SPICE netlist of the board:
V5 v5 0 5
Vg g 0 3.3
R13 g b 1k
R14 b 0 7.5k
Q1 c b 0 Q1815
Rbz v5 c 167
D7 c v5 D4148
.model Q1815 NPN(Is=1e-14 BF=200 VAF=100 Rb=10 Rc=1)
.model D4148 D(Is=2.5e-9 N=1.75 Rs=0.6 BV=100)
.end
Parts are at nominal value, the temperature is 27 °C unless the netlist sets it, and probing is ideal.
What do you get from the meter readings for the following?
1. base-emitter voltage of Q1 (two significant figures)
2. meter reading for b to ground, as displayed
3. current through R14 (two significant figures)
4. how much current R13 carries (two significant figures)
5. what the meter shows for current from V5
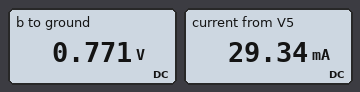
770 mV
0.771 V
100 µA
2.5 mA
29.34 mA
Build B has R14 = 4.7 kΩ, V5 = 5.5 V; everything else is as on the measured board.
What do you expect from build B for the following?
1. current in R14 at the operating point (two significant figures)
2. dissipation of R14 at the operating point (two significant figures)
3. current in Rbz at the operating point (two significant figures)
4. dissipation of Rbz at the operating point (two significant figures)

160 µA
130 µW
32 mA
170 mW
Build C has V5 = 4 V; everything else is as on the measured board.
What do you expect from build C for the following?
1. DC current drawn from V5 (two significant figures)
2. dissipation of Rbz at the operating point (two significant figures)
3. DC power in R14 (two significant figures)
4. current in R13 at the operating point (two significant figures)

23 mA
92 mW
78 µW
2.5 mA
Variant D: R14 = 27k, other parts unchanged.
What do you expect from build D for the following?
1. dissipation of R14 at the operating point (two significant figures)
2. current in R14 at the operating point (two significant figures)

22 µW
29 µA
